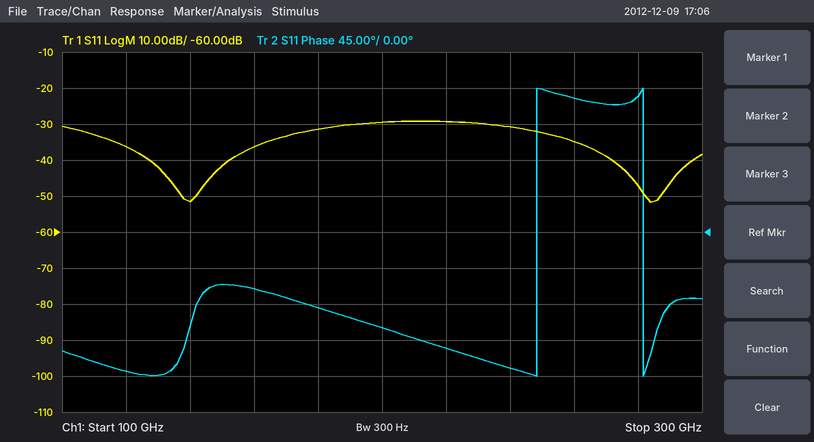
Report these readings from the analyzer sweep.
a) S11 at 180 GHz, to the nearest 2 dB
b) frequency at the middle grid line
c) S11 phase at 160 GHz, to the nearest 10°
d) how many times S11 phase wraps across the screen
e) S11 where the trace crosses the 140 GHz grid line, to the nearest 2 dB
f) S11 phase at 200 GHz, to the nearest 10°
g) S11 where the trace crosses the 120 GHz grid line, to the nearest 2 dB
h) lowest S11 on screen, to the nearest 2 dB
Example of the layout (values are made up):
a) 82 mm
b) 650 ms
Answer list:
a) -32 dB
b) 200 GHz
c) -70°
d) 2
e) -52 dB
f) -120°
g) -36 dB
h) -52 dB
